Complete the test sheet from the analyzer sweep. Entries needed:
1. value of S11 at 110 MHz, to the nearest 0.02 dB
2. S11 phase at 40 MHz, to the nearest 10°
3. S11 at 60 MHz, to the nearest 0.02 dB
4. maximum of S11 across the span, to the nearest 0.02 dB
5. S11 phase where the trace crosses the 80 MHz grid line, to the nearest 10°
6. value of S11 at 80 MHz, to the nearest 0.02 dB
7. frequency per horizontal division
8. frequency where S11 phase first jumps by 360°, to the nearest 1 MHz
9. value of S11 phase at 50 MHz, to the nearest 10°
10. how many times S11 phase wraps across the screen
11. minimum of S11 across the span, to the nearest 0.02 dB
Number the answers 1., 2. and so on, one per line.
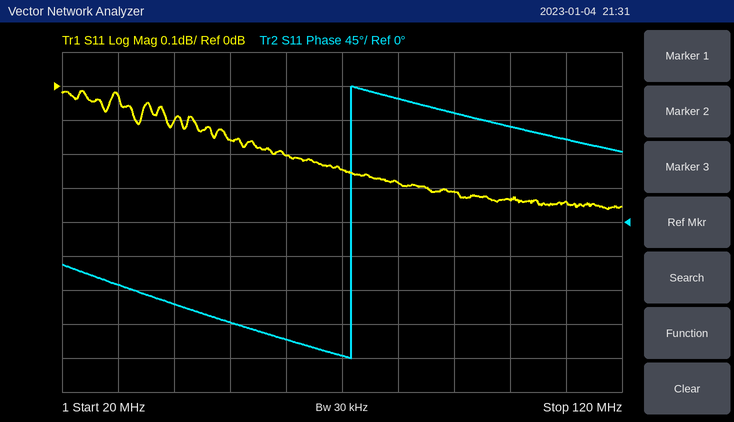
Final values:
1. -0.34 dB
2. -110°
3. -0.20 dB
4. -0.02 dB
5. 160°
6. -0.28 dB
7. 10 MHz
8. 72 MHz
9. -130°
10. 1
11. -0.36 dB
